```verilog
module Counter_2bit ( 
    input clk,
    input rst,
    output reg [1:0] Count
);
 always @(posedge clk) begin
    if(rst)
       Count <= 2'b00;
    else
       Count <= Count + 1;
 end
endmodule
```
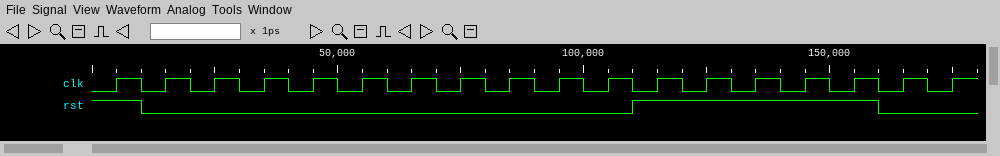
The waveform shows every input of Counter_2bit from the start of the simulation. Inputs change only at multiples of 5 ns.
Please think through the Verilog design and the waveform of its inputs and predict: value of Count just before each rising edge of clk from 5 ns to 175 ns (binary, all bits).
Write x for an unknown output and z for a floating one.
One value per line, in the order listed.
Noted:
x, 00, 01, 10, 11, 00, 01, 10, 11, 00, 01, 10, 00, 00, 00, 00, 00, 01
